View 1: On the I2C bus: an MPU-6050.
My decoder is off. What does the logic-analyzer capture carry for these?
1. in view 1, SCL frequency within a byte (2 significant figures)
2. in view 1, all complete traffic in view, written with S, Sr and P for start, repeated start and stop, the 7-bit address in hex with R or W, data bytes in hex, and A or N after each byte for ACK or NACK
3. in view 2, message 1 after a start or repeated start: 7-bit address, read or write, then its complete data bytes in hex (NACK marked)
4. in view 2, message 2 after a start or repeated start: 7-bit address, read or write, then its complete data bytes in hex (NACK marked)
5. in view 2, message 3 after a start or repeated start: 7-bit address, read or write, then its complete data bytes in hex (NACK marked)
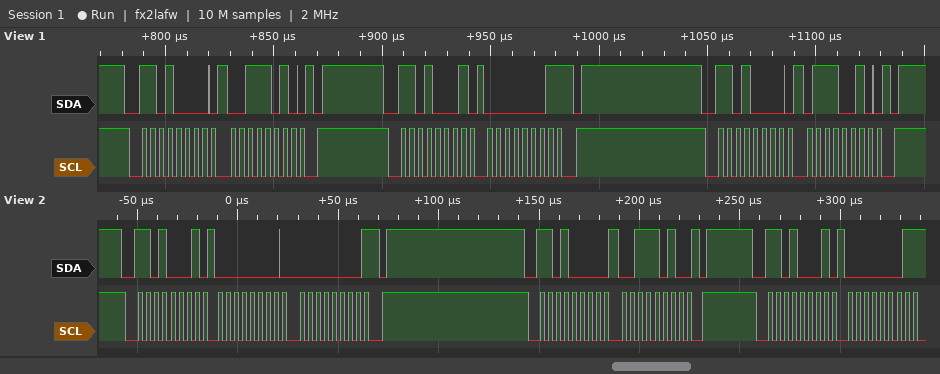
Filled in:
250 kHz
S 68W A 3A A P S 68R A 01 N P S 68W A 72 A P
0x68 read: 00 00 NACK
0x68 write: 3A
0x68 read: 01 NACK
